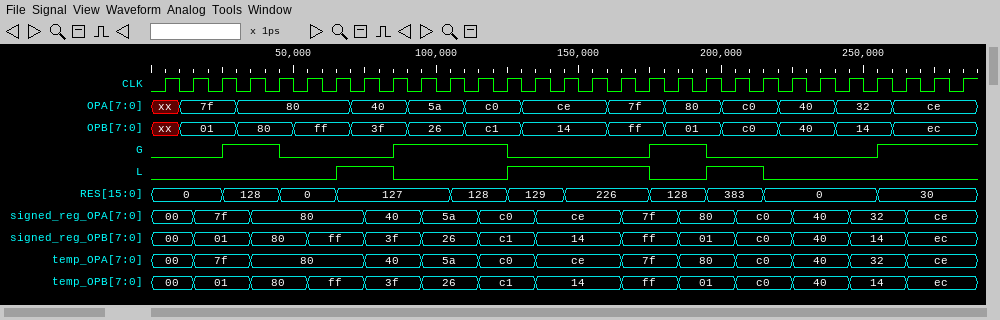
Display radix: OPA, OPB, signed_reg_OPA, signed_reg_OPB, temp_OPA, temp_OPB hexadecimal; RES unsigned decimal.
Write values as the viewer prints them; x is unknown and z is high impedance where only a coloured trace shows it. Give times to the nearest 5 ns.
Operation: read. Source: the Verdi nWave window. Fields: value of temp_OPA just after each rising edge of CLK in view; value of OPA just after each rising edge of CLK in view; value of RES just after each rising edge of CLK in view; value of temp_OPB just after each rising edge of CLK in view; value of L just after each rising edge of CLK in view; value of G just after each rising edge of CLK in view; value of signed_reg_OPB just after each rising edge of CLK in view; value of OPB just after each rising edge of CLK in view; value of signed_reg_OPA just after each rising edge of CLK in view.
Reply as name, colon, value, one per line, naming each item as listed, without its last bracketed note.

value of temp_OPA just after each rising edge of CLK in view: 00, 7f, 7f, 80, 80, 80, 80, 40, 40, 5a, 5a, c0, c0, ce, ce, ce, 7f, 7f, 80, 80, c0, c0, 40, 40, 32, 32, ce, ce, ce
value of OPA just after each rising edge of CLK in view: xx, 7f, 7f, 80, 80, 80, 80, 40, 40, 5a, 5a, c0, c0, ce, ce, ce, 7f, 7f, 80, 80, c0, c0, 40, 40, 32, 32, ce, ce, ce
value of RES just after each rising edge of CLK in view: 0, 0, 128, 128, 0, 0, 127, 127, 127, 127, 128, 128, 129, 129, 226, 226, 226, 128, 128, 383, 383, 0, 0, 0, 0, 30, 30, 30, 30
value of temp_OPB just after each rising edge of CLK in view: 00, 01, 01, 80, 80, ff, ff, 3f, 3f, 26, 26, c1, c1, 14, 14, 14, ff, ff, 01, 01, c0, c0, 40, 40, 14, 14, ec, ec, ec
value of L just after each rising edge of CLK in view: 0 0 0 0 0 0 1 1 0 0 0 0 1 1 1 1 1 0 0 1 1 0 0 0 0 0 0 0 0
value of G just after each rising edge of CLK in view: 0 0 1 1 0 0 0 0 1 1 1 1 0 0 0 0 0 1 1 0 0 0 0 0 0 1 1 1 1
value of signed_reg_OPB just after each rising edge of CLK in view: 00, 01, 01, 80, 80, ff, ff, 3f, 3f, 26, 26, c1, c1, 14, 14, 14, ff, ff, 01, 01, c0, c0, 40, 40, 14, 14, ec, ec, ec
value of OPB just after each rising edge of CLK in view: xx, 01, 01, 80, 80, ff, ff, 3f, 3f, 26, 26, c1, c1, 14, 14, 14, ff, ff, 01, 01, c0, c0, 40, 40, 14, 14, ec, ec, ec
value of signed_reg_OPA just after each rising edge of CLK in view: 00, 7f, 7f, 80, 80, 80, 80, 40, 40, 5a, 5a, c0, c0, ce, ce, ce, 7f, 7f, 80, 80, c0, c0, 40, 40, 32, 32, ce, ce, ce
